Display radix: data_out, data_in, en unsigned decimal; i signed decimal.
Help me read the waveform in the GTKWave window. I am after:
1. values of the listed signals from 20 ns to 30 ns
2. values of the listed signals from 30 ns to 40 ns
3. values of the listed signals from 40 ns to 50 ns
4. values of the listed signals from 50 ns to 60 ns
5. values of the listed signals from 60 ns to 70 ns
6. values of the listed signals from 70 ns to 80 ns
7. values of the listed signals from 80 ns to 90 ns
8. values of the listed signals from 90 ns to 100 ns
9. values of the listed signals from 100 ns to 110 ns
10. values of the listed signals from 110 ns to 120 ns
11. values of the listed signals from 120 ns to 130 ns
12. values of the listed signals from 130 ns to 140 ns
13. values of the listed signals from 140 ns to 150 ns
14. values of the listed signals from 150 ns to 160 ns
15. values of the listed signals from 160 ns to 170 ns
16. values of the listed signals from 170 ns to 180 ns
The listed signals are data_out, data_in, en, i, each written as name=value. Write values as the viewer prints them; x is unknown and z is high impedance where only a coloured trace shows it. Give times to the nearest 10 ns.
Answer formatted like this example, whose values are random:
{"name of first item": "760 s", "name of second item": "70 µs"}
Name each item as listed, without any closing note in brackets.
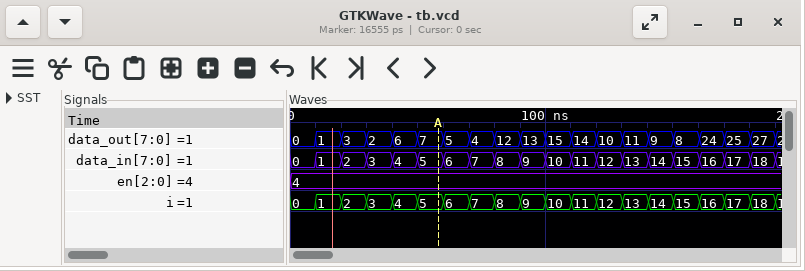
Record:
{"values of the listed signals from 20 ns to 30 ns": "data_out=3, data_in=2, en=4, i=2", "values of the listed signals from 30 ns to 40 ns": "data_out=2, data_in=3, en=4, i=3", "values of the listed signals from 40 ns to 50 ns": "data_out=6, data_in=4, en=4, i=4", "values of the listed signals from 50 ns to 60 ns": "data_out=7, data_in=5, en=4, i=5", "values of the listed signals from 60 ns to 70 ns": "data_out=5, data_in=6, en=4, i=6", "values of the listed signals from 70 ns to 80 ns": "data_out=4, data_in=7, en=4, i=7", "values of the listed signals from 80 ns to 90 ns": "data_out=12, data_in=8, en=4, i=8", "values of the listed signals from 90 ns to 100 ns": "data_out=13, data_in=9, en=4, i=9", "values of the listed signals from 100 ns to 110 ns": "data_out=15, data_in=10, en=4, i=10", "values of the listed signals from 110 ns to 120 ns": "data_out=14, data_in=11, en=4, i=11", "values of the listed signals from 120 ns to 130 ns": "data_out=10, data_in=12, en=4, i=12", "values of the listed signals from 130 ns to 140 ns": "data_out=11, data_in=13, en=4, i=13", "values of the listed signals from 140 ns to 150 ns": "data_out=9, data_in=14, en=4, i=14", "values of the listed signals from 150 ns to 160 ns": "data_out=8, data_in=15, en=4, i=15", "values of the listed signals from 160 ns to 170 ns": "data_out=24, data_in=16, en=4, i=16", "values of the listed signals from 170 ns to 180 ns": "data_out=25, data_in=17, en=4, i=17"}
